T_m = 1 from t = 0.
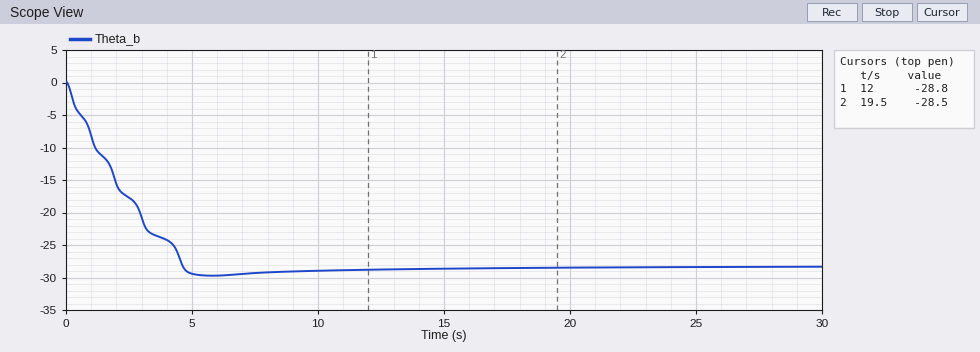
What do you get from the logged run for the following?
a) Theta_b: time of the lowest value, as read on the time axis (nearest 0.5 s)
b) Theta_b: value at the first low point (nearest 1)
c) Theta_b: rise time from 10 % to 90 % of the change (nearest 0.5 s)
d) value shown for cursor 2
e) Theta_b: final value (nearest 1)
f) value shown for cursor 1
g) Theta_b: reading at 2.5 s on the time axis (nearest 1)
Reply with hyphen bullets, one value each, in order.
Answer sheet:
- 6.0 s
- -30
- 4.0 s
- -28.5
- -28
- -28.8
- -18
